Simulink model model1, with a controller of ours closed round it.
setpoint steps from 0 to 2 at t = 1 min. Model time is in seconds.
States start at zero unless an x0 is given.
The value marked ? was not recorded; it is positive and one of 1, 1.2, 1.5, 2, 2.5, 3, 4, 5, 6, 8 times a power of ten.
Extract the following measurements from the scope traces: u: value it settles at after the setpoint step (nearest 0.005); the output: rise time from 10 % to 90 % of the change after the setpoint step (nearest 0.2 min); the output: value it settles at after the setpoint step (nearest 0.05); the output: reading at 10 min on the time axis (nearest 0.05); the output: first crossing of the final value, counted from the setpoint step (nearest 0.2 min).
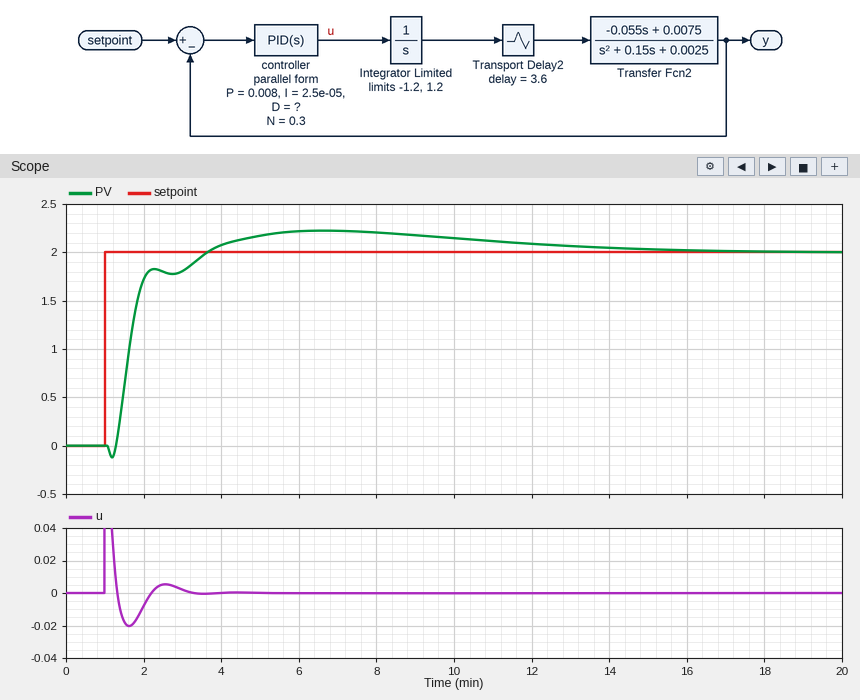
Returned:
0.000
0.8 min
2.00
2.15
2.6 min
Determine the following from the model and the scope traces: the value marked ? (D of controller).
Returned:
0.6
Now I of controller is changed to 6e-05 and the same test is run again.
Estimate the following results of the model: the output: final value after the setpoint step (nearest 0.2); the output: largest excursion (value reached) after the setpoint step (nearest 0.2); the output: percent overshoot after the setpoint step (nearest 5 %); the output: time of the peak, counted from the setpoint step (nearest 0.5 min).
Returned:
2.0
2.4
20 %
4.0 min
